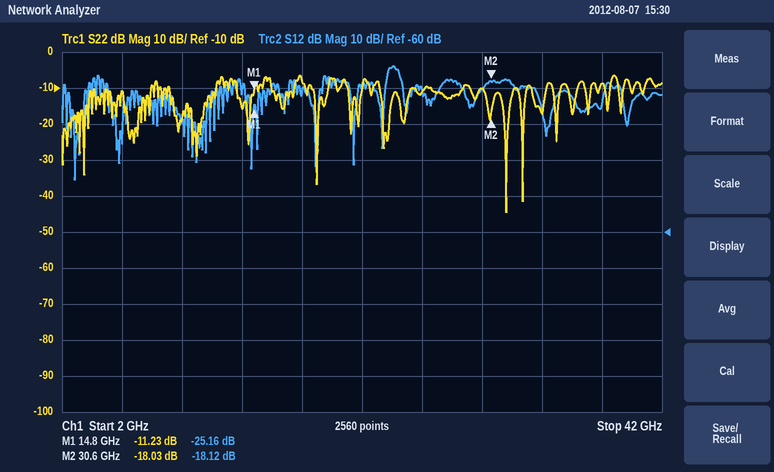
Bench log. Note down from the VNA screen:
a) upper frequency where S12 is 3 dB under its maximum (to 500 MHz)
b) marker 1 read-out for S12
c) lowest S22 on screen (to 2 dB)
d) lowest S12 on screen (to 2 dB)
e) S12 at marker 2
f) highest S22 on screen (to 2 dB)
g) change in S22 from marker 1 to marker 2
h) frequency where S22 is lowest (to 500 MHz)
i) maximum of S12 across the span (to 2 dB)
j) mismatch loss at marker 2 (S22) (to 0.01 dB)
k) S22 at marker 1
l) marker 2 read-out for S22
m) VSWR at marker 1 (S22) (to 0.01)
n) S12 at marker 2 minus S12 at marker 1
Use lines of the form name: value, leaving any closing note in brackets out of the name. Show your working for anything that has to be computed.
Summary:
upper frequency where S12 is 3 dB under its maximum: 24.5 GHz
marker 1 read-out for S12: -25.16 dB
lowest S22 on screen: -44 dB
lowest S12 on screen: -46 dB
S12 at marker 2: -18.12 dB
highest S22 on screen: -6 dB
change in S22 from marker 1 to marker 2: -18.03 − (-11.23) = -6.80 dB
frequency where S22 is lowest: 31.5 GHz
maximum of S12 across the span: -14 dB
mismatch loss at marker 2 (S22): −10 log10(1 − 10^(-18.03/10)) ≈ 0.07 dB
S22 at marker 1: -11.23 dB
marker 2 read-out for S22: -18.03 dB
VSWR at marker 1 (S22): (1 + 0.2745)/(1 − 0.2745) ≈ 1.76
S12 at marker 2 minus S12 at marker 1: -18.12 − (-25.16) = 7.04 dB
